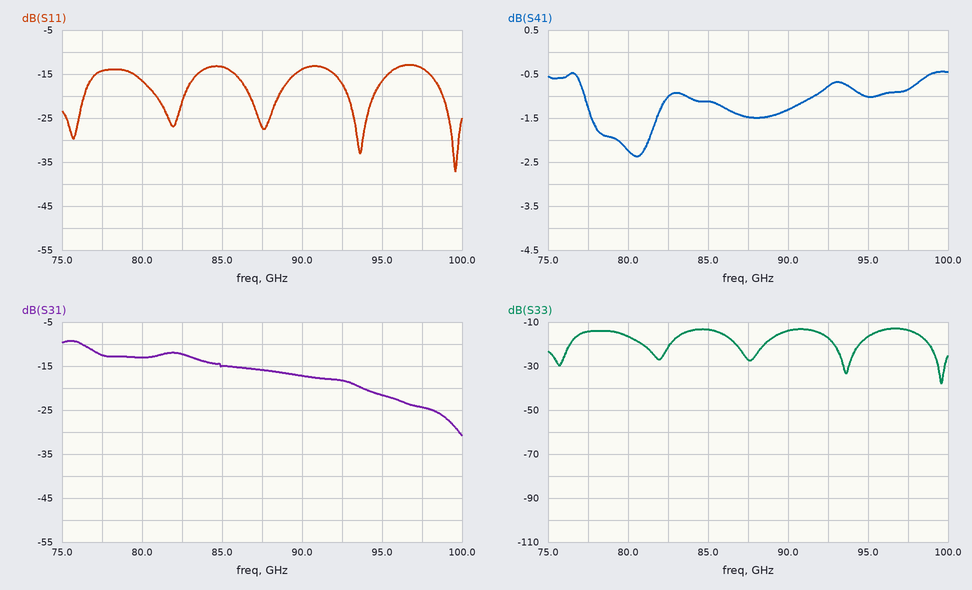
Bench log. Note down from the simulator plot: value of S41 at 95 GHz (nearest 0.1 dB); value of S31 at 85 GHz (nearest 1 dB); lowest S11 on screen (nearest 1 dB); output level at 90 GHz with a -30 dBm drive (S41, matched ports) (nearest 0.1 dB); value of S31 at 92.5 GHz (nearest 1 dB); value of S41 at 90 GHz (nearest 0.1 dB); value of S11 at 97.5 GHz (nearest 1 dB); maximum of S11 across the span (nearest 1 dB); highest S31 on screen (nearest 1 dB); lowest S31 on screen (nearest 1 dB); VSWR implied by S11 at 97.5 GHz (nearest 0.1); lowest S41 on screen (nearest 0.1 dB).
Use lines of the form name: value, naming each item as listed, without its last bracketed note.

value of S41 at 95 GHz: -1.0 dB
value of S31 at 85 GHz: -15 dB
lowest S11 on screen: -37 dB
output level at 90 GHz with a -30 dBm drive (S41, matched ports): -31.3 dBm
value of S31 at 92.5 GHz: -18 dB
value of S41 at 90 GHz: -1.3 dB
value of S11 at 97.5 GHz: -14 dB
maximum of S11 across the span: -13 dB
highest S31 on screen: -9 dB
lowest S31 on screen: -31 dB
VSWR implied by S11 at 97.5 GHz: 1.5
lowest S41 on screen: -2.4 dB
